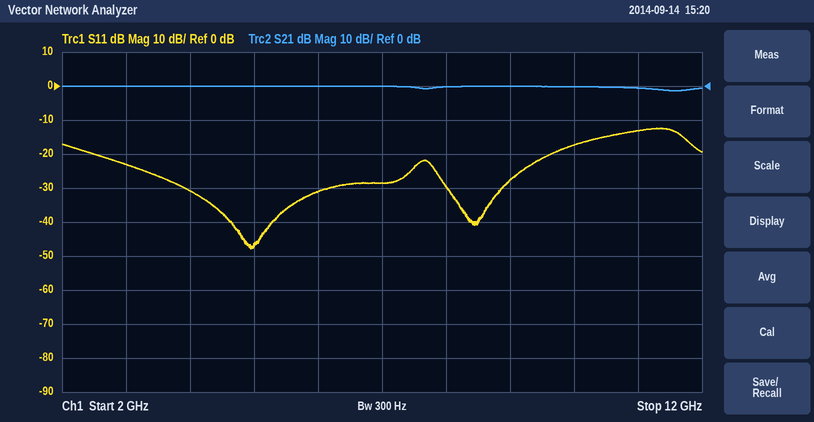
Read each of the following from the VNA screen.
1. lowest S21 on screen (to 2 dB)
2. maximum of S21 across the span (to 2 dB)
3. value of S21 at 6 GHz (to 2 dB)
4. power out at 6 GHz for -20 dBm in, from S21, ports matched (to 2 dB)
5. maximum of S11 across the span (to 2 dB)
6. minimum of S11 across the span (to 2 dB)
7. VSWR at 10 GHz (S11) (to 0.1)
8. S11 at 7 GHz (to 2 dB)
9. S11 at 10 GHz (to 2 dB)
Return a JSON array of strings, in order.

["-2 dB", "0 dB", "0 dB", "-20 dBm", "-12 dB", "-48 dB", "1.3", "-28 dB", "-18 dB"]
